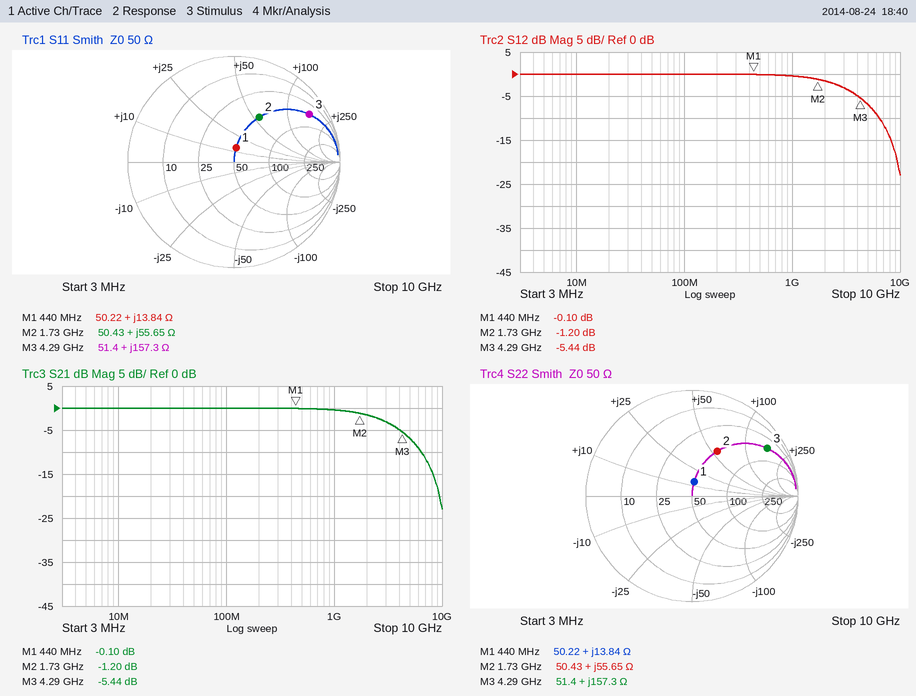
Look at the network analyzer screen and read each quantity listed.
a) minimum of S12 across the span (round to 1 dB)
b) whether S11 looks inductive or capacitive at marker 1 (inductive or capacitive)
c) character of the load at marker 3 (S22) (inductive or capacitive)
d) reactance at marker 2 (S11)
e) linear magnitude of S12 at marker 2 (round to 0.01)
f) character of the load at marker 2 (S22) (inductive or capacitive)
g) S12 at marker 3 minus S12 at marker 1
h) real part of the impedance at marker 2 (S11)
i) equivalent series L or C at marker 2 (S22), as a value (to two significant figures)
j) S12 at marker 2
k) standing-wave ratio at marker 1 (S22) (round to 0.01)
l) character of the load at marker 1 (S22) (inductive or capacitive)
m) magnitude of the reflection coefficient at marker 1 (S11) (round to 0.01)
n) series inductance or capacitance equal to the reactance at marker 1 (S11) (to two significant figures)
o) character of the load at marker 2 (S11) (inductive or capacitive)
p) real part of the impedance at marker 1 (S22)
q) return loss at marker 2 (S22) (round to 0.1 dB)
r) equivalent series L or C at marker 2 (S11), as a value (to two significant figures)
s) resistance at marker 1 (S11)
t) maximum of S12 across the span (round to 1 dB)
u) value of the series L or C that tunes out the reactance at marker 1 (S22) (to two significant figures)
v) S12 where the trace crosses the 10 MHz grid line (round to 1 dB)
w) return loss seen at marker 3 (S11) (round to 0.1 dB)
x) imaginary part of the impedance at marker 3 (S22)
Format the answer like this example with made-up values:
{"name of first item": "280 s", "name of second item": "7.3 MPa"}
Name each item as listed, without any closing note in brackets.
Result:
{"minimum of S12 across the span": "-23 dB", "whether S11 looks inductive or capacitive at marker 1": "inductive", "character of the load at marker 3 (S22)": "inductive", "reactance at marker 2": "+55.65 Ω", "linear magnitude of S12 at marker 2": "0.87", "character of the load at marker 2 (S22)": "inductive", "S12 at marker 3 minus S12 at marker 1": "-5.34 dB", "real part of the impedance at marker 2": "50.43 Ω", "equivalent series L or C at marker 2 (S22), as a value": "5.1 nH", "S12 at marker 2": "-1.20 dB", "standing-wave ratio at marker 1 (S22)": "1.32", "character of the load at marker 1 (S22)": "inductive", "magnitude of the reflection coefficient at marker 1 (S11)": "0.14", "series inductance or capacitance equal to the reactance at marker 1 (S11)": "5.0 nH", "character of the load at marker 2 (S11)": "inductive", "real part of the impedance at marker 1": "50.22 Ω", "return loss at marker 2 (S22)": "6.3 dB", "equivalent series L or C at marker 2 (S11), as a value": "5.1 nH", "resistance at marker 1": "50.22 Ω", "maximum of S12 across the span": "0 dB", "value of the series L or C that tunes out the reactance at marker 1 (S22)": "26 pF", "S12 where the trace crosses the 10 MHz grid line": "0 dB", "return loss seen at marker 3 (S11)": "1.5 dB", "imaginary part of the impedance at marker 3": "+157.3 Ω"}
